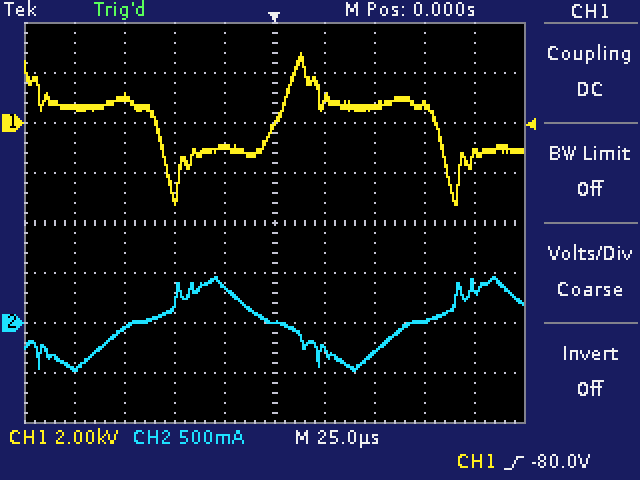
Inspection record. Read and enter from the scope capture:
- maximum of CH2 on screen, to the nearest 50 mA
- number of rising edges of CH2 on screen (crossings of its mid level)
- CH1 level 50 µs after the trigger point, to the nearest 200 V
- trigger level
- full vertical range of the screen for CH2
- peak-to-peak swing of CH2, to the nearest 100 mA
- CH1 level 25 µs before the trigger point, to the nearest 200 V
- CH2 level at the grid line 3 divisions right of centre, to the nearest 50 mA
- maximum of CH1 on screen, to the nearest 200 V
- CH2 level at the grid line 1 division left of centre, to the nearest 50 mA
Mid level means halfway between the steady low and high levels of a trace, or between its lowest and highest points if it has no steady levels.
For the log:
450 mA
2
600 V
-80.0 V
4 A
900 mA
-1.0 kV
0 mA
2.8 kV
350 mA
